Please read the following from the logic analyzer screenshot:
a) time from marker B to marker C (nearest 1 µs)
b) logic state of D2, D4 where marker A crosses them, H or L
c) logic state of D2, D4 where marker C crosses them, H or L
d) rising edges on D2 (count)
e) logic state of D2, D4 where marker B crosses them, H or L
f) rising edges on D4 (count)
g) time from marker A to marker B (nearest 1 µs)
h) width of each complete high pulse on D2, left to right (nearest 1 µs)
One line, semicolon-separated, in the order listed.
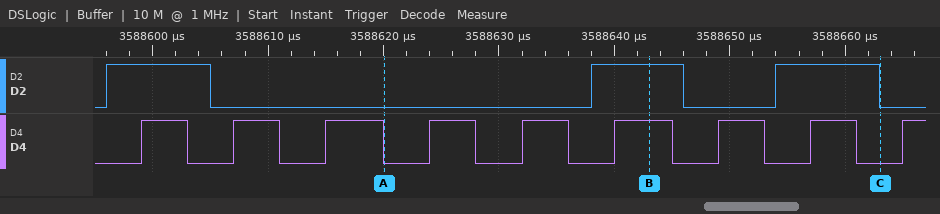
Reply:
20 µs; D2=L, D4=L; D2=L, D4=L; 3; D2=H, D4=H; 9; 23 µs; 9 µs, 8 µs, 9 µs
